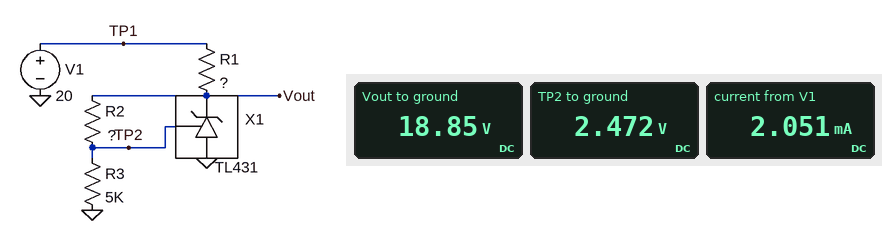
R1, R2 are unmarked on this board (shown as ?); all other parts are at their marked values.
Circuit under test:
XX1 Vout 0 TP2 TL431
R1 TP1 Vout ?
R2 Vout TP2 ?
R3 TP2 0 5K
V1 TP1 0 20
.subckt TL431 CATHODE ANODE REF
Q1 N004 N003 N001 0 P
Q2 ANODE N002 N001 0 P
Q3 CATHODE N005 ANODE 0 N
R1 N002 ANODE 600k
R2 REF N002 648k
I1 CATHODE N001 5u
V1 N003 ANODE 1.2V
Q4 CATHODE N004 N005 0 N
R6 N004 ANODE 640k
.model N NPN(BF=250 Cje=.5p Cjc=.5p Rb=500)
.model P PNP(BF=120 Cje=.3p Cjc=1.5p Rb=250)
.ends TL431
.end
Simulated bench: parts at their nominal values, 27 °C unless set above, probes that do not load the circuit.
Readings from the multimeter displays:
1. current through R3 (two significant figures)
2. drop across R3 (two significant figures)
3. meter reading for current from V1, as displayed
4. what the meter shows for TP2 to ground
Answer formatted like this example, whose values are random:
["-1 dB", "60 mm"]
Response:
["490 µA", "2.5 V", "2.051 mA", "2.472 V"]
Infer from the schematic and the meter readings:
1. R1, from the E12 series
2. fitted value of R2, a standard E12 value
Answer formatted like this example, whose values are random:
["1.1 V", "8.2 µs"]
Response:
["560 Ω", "33 kΩ"]
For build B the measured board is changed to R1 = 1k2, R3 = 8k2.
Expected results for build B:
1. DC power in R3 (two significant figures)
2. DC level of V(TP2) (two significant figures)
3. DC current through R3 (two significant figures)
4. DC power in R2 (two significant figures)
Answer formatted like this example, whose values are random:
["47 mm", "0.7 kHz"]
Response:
["750 µW", "2.5 V", "300 µA", "3.1 mW"]
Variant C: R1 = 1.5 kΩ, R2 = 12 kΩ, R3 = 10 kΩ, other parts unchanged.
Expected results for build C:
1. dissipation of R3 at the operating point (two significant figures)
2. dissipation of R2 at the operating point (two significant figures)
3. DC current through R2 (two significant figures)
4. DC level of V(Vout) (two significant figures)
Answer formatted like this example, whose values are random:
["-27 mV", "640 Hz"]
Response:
["620 µW", "750 µW", "250 µA", "5.5 V"]
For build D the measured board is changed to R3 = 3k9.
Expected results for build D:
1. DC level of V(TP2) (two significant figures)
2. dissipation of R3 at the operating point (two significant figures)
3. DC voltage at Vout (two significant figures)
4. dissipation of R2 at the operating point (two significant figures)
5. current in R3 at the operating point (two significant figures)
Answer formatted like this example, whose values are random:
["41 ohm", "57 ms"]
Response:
["2.1 V", "1.1 mW", "20 V", "9.4 mW", "530 µA"]
